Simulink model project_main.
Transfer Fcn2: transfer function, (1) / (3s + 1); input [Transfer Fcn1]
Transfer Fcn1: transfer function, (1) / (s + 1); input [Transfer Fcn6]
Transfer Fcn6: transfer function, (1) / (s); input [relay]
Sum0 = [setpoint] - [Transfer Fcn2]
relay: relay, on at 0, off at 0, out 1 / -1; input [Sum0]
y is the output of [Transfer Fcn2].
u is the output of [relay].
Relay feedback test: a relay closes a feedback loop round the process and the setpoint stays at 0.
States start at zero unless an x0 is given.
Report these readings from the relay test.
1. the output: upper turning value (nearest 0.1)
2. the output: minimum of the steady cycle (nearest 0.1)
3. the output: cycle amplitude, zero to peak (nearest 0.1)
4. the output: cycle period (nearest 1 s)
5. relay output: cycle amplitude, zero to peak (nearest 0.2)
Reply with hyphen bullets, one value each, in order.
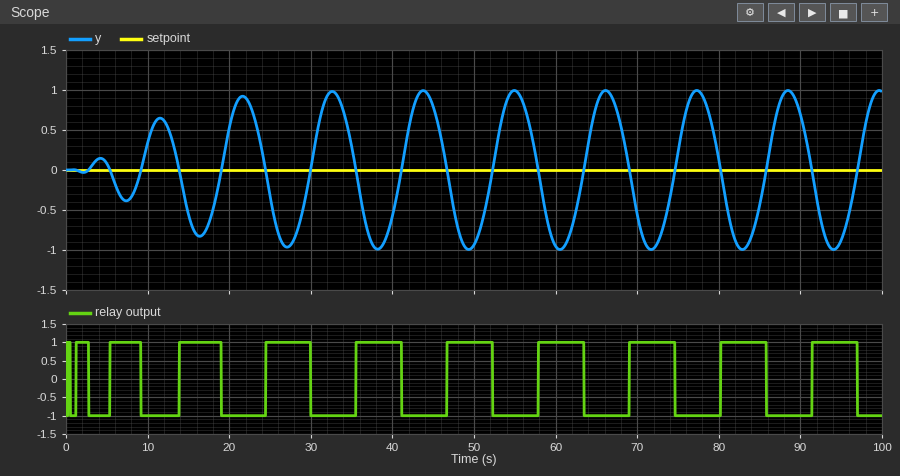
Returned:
- 1.0
- -1.0
- 1.0
- 11 s
- 1.0
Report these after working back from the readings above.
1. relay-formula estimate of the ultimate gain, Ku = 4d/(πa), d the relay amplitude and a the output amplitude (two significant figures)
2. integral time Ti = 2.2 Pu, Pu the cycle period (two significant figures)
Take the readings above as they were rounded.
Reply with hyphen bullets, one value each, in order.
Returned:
- 1.3
- 24 s
